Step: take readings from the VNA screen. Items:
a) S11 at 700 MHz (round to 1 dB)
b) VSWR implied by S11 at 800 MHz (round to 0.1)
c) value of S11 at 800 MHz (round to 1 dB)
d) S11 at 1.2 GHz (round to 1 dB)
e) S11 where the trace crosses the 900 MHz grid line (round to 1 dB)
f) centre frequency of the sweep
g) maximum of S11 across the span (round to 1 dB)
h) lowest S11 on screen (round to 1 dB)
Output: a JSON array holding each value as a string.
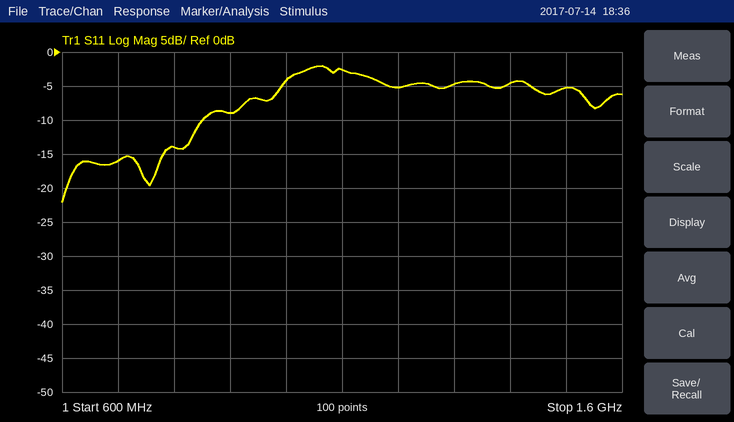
["-16 dB", "1.5", "-14 dB", "-5 dB", "-9 dB", "1.1 GHz", "-2 dB", "-22 dB"]
